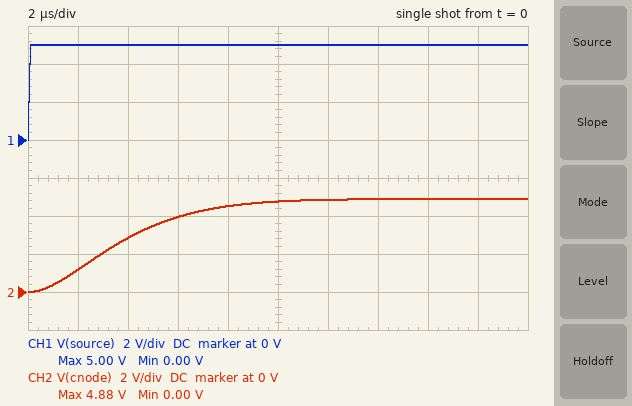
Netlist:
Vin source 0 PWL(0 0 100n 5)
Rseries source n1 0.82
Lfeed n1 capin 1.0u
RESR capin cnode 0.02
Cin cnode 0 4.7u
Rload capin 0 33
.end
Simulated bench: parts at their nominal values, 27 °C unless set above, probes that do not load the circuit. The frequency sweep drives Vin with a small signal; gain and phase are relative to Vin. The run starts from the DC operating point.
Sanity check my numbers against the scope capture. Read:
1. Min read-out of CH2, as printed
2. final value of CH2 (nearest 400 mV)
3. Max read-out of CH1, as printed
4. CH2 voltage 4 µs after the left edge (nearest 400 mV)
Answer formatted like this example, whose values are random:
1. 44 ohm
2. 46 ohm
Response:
1. 0.00 V
2. 4.8 V
3. 5.00 V
4. 2.8 V
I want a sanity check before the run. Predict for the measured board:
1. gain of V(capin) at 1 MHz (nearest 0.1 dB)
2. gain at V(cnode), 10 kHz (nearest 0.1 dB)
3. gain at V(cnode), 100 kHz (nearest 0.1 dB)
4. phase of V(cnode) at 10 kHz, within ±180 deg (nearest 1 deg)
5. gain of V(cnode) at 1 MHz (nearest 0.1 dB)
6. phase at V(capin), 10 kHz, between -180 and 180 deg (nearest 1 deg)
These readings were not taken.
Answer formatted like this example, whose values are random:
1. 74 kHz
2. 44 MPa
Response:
1. -44.1 dB
2. -0.3 dB
3. -8.4 dB
4. -14 deg
5. -45.4 dB
6. -14 deg
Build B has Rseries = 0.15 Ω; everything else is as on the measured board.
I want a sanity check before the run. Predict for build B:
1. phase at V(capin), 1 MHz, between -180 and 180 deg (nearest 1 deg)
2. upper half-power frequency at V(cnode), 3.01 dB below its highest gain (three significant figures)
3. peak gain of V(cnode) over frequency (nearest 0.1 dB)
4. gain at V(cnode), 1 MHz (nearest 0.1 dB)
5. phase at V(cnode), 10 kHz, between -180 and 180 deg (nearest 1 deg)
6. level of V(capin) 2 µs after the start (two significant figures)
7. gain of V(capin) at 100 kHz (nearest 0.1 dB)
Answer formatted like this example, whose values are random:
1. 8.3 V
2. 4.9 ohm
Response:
1. -148 deg
2. 83.9 kHz
3. 8.5 dB
4. -45.3 dB
5. -3 deg
6. 1.8 V
7. 0 dB
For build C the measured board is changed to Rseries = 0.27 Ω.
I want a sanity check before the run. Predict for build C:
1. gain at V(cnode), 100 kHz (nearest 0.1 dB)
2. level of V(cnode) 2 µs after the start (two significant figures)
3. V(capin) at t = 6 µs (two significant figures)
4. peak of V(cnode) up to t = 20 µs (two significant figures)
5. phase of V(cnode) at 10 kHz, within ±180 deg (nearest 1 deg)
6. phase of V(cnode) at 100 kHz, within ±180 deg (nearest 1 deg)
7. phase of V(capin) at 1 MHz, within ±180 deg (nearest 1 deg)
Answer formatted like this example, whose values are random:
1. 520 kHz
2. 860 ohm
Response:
1. -1.7 dB
2. 1.6 V
3. 6.4 V
4. 6.7 V
5. -5 deg
6. -134 deg
7. -147 deg
